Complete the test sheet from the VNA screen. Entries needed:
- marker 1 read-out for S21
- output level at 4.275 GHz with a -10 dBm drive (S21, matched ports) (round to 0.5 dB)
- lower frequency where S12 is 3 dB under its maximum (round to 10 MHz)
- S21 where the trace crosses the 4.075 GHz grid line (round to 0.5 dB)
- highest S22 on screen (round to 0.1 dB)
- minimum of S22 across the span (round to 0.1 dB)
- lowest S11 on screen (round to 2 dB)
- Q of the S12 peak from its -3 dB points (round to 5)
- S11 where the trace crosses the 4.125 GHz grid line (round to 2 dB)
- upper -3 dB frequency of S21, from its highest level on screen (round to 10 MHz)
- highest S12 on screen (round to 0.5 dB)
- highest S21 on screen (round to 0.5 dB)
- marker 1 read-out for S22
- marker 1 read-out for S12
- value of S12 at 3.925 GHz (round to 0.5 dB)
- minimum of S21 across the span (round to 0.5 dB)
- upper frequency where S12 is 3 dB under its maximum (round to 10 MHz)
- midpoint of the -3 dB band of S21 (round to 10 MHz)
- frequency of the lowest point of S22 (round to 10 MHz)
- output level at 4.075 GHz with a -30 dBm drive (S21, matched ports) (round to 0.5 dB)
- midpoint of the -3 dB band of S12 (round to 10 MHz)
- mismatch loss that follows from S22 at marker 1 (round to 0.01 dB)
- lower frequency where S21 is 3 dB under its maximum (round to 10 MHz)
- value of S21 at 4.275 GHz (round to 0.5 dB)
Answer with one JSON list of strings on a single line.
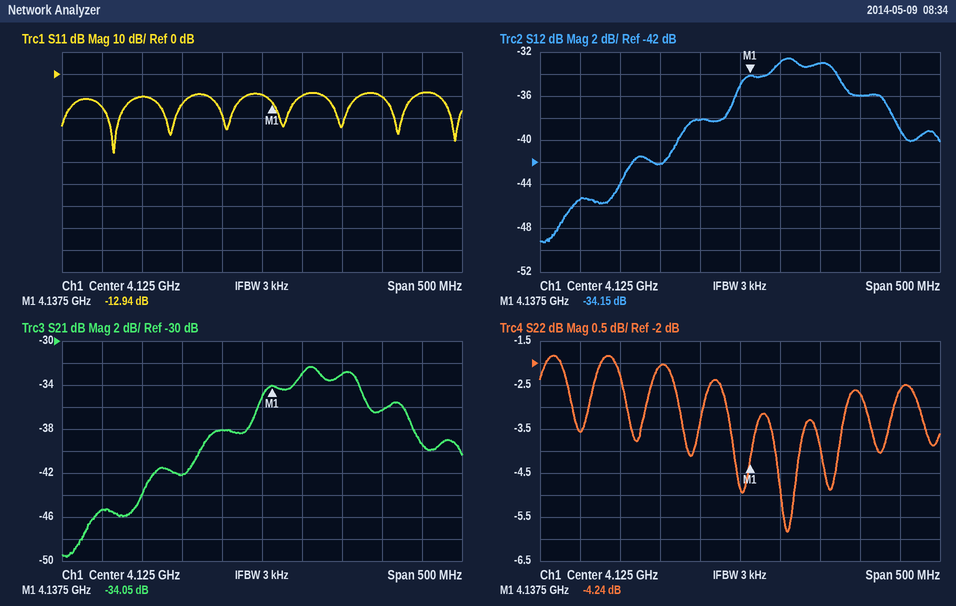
["-34.05 dB", "-46.5 dBm", "4.12 GHz", "-38.0 dB", "-1.8 dB", "-5.8 dB", "-36 dB", "30", "-10 dB", "4.25 GHz", "-32.5 dB", "-32.5 dB", "-4.24 dB", "-34.15 dB", "-45.5 dB", "-49.5 dB", "4.26 GHz", "4.19 GHz", "4.18 GHz", "-68.0 dBm", "4.19 GHz", "2.05 dB", "4.12 GHz", "-36.5 dB"]
